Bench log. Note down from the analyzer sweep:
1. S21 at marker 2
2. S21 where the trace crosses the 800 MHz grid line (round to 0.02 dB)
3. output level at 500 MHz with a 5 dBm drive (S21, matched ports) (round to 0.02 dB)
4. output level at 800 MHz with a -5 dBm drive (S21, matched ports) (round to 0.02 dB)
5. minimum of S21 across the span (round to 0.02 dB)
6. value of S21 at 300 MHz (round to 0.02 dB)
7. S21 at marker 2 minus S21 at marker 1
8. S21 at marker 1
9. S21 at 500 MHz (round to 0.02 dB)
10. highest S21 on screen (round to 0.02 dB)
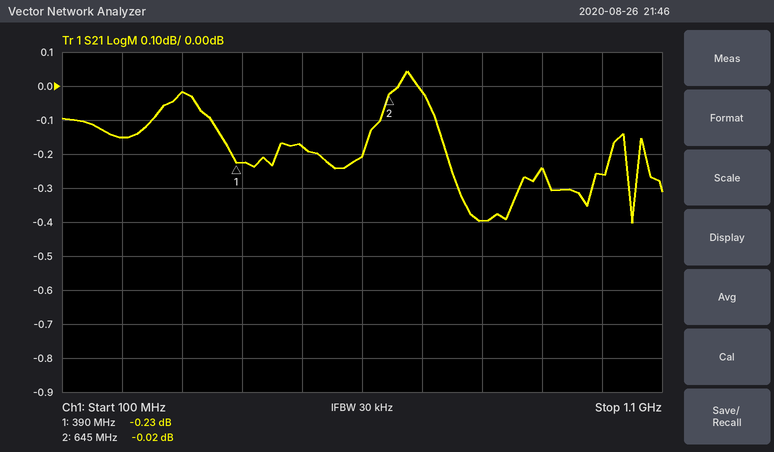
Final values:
-0.02 dB
-0.40 dB
4.82 dBm
-5.40 dBm
-0.40 dB
-0.02 dB
0.21 dB
-0.23 dB
-0.18 dB
0.04 dB
